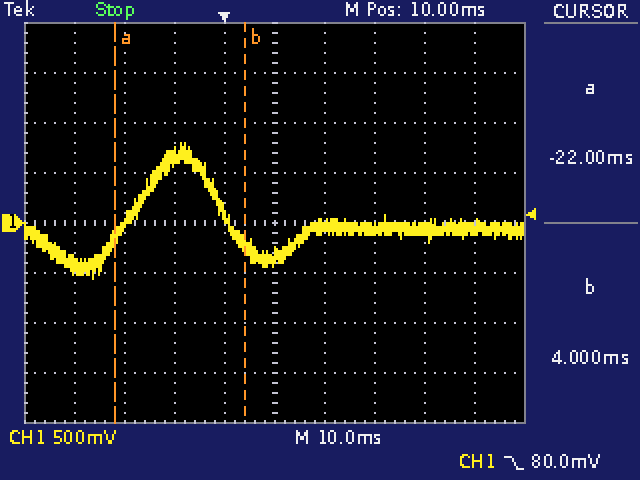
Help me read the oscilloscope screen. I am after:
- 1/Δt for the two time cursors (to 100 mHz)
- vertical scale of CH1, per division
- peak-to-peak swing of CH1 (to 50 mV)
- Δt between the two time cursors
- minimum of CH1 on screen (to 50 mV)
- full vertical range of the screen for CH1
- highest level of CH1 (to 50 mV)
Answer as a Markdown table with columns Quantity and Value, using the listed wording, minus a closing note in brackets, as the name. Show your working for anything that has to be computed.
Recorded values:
| Quantity | Value |
|---|---|
| 1/Δt for the two time cursors | 1 / 26 ms ≈ 38.5 Hz |
| vertical scale of CH1, per division | 500 mV |
| peak-to-peak swing of CH1 | 800 mV − (-550 mV) = 1.35 V |
| Δt between the two time cursors | 4 ms − (-22 ms) = 26 ms |
| minimum of CH1 on screen | -550 mV |
| full vertical range of the screen for CH1 | 4 V |
| highest level of CH1 | 800 mV |
